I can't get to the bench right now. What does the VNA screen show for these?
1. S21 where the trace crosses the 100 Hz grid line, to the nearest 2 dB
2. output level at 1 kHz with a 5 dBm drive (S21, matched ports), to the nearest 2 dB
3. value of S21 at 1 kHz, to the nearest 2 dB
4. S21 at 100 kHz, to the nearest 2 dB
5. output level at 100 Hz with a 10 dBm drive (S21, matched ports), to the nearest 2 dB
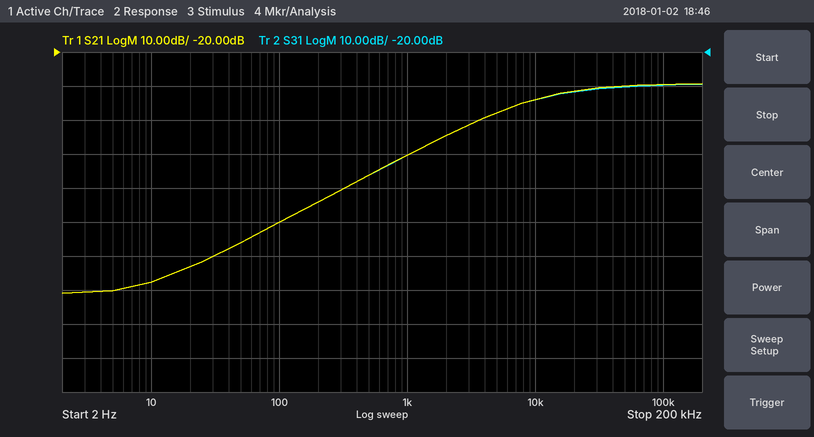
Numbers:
-70 dB
-46 dBm
-50 dB
-30 dB
-60 dBm
